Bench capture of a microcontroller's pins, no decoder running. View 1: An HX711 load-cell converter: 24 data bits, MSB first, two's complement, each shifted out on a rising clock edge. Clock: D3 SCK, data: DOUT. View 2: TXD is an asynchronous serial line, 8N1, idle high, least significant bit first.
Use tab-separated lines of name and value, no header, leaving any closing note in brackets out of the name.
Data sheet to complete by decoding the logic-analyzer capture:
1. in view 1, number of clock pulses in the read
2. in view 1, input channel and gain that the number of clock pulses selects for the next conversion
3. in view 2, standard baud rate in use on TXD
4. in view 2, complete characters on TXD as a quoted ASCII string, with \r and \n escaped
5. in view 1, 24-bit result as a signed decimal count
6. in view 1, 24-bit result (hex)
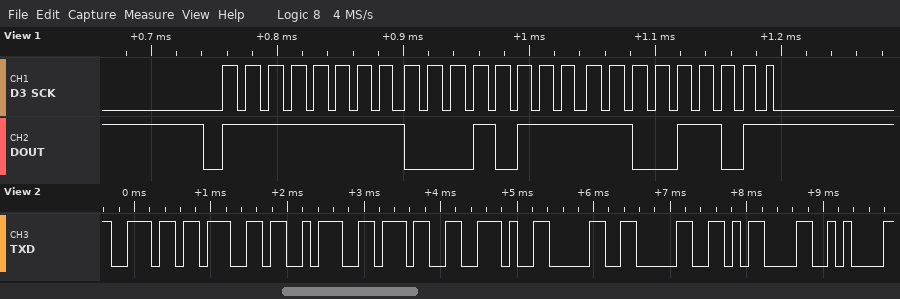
in view 1, number of clock pulses in the read	25
in view 1, input channel and gain that the number of clock pulses selects for the next conversion	channel A, gain 128
in view 2, standard baud rate in use on TXD	9600 baud
in view 2, complete characters on TXD as a quoted ASCII string, with \r and \n escaped	"ng:7.00\r\n"
in view 1, 24-bit result as a signed decimal count	-59443
in view 1, 24-bit result	0xFF17CD
